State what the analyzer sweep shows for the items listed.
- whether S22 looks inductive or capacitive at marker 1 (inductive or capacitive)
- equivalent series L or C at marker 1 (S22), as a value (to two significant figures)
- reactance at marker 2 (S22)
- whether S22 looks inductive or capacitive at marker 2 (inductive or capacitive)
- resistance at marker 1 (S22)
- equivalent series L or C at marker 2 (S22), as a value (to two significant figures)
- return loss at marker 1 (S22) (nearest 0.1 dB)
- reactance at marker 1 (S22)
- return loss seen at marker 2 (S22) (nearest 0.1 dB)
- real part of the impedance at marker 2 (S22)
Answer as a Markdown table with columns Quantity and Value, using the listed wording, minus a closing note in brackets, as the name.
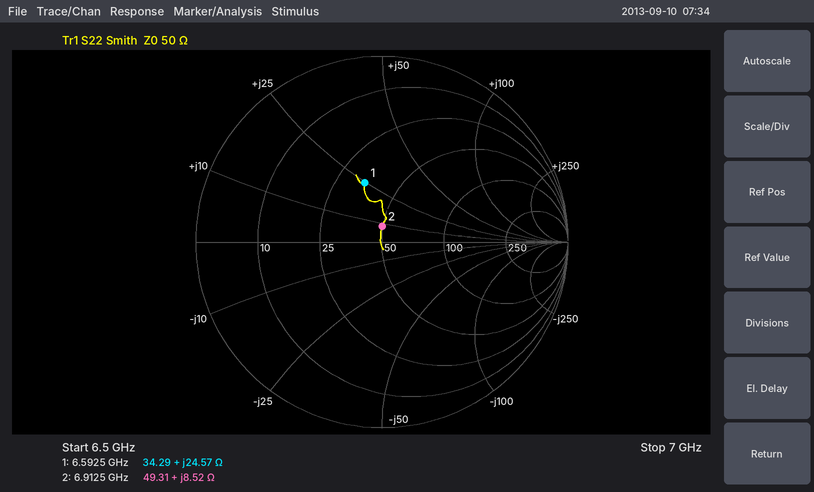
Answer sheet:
| Quantity | Value |
|---|---|
| whether S22 looks inductive or capacitive at marker 1 | inductive |
| equivalent series L or C at marker 1 (S22), as a value | 590 pH |
| reactance at marker 2 | +8.52 Ω |
| whether S22 looks inductive or capacitive at marker 2 | inductive |
| resistance at marker 1 | 34.29 Ω |
| equivalent series L or C at marker 2 (S22), as a value | 200 pH |
| return loss at marker 1 (S22) | 9.6 dB |
| reactance at marker 1 | +24.57 Ω |
| return loss seen at marker 2 (S22) | 21.3 dB |
| real part of the impedance at marker 2 | 49.31 Ω |
